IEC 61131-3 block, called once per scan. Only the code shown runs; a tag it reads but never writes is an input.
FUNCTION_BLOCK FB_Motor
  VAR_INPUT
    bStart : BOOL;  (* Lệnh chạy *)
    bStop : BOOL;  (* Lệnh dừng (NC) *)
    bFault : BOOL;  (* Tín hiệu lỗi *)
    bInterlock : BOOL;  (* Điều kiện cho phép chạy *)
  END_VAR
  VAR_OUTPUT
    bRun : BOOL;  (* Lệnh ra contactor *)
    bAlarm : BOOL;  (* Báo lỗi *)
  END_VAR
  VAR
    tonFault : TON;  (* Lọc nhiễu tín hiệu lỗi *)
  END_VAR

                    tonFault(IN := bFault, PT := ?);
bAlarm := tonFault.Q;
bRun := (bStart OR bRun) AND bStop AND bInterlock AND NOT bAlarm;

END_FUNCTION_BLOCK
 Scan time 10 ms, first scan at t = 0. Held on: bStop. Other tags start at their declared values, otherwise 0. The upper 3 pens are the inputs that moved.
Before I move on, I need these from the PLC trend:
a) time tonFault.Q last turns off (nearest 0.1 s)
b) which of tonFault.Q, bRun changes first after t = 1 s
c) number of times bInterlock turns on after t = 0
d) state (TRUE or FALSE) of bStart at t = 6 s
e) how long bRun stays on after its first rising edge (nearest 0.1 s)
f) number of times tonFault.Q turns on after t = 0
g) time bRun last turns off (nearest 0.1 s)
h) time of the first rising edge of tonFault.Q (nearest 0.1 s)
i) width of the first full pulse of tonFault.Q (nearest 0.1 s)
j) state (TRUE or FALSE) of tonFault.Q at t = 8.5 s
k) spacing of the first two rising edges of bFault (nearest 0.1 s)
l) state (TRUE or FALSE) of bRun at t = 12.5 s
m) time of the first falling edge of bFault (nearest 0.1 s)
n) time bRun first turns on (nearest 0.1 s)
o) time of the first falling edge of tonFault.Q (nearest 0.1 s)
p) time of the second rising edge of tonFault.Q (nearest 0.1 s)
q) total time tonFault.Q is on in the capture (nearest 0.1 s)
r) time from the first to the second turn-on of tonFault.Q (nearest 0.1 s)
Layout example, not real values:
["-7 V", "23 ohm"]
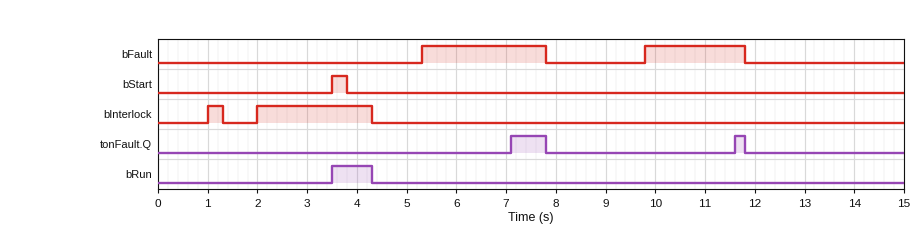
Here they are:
["11.8 s", "bRun", "2", "FALSE", "0.8 s", "2", "4.3 s", "7.1 s", "0.7 s", "FALSE", "4.5 s", "FALSE", "7.8 s", "3.5 s", "7.8 s", "11.6 s", "0.9 s", "4.5 s"]
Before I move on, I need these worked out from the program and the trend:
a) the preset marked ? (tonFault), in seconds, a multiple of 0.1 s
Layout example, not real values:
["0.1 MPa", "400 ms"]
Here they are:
["1.8 s"]
